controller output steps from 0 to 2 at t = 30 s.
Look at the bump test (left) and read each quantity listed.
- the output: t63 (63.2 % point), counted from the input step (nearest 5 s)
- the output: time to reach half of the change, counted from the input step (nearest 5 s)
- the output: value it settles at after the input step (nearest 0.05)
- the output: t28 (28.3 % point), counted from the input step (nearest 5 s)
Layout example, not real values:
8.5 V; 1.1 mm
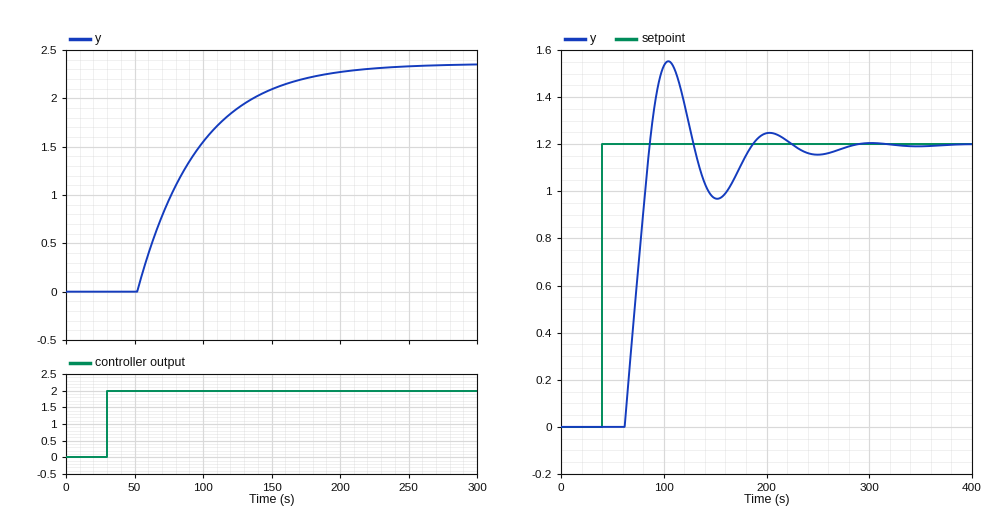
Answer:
65 s; 55 s; 2.35; 35 s
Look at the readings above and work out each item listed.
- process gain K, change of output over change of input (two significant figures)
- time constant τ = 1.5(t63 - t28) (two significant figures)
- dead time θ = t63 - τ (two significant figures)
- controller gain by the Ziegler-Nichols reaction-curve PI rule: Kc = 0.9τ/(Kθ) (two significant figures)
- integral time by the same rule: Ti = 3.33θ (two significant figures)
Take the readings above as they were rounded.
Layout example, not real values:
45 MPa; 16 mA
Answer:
1.2; 45 s; 20 s; 1.7; 67 s
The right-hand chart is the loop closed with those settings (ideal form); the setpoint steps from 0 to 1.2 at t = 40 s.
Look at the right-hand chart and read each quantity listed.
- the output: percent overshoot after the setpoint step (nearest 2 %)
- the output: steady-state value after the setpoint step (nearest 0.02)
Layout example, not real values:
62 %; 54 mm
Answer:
30 %; 1.20
